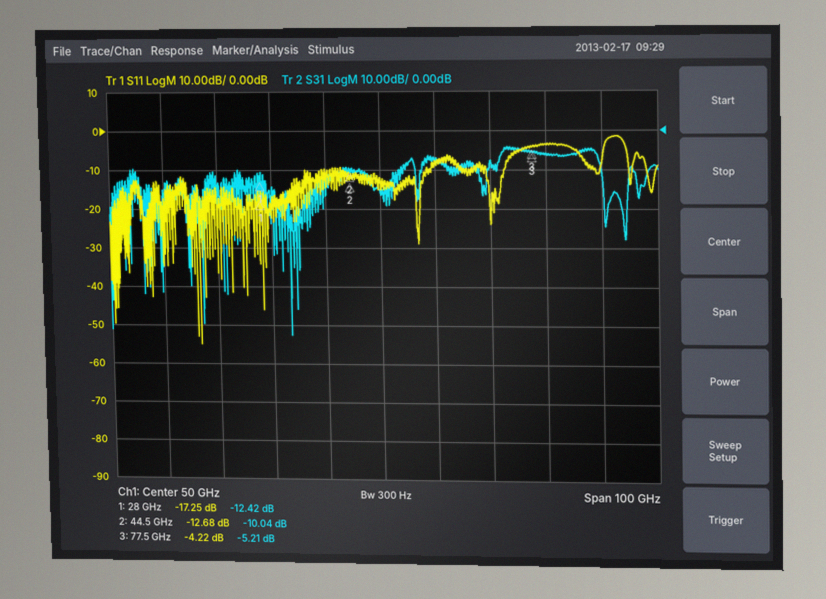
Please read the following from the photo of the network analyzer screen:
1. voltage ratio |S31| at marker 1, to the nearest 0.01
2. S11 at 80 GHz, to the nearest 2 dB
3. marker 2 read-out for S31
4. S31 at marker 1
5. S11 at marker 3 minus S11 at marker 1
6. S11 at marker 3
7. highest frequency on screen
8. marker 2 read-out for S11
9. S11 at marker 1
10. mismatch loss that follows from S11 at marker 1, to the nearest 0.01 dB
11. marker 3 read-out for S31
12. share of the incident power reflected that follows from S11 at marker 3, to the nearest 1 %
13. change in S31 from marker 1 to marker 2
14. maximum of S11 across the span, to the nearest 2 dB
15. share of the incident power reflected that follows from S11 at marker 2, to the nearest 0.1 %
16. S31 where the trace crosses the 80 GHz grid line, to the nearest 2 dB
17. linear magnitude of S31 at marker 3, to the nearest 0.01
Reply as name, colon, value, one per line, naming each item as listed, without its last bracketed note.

voltage ratio |S31| at marker 1, to the nearest 0.01: 0.24
S11 at 80 GHz, to the nearest 2 dB: -4 dB
marker 2 read-out for S31: -10.04 dB
S31 at marker 1: -12.42 dB
S11 at marker 3 minus S11 at marker 1: 13.03 dB
S11 at marker 3: -4.22 dB
highest frequency on screen: 100 GHz
marker 2 read-out for S11: -12.68 dB
S11 at marker 1: -17.25 dB
mismatch loss that follows from S11 at marker 1, to the nearest 0.01 dB: 0.08 dB
marker 3 read-out for S31: -5.21 dB
share of the incident power reflected that follows from S11 at marker 3, to the nearest 1 %: 38 %
change in S31 from marker 1 to marker 2: 2.38 dB
maximum of S11 across the span, to the nearest 2 dB: -2 dB
share of the incident power reflected that follows from S11 at marker 2, to the nearest 0.1 %: 5.4 %
S31 where the trace crosses the 80 GHz grid line, to the nearest 2 dB: -6 dB
linear magnitude of S31 at marker 3, to the nearest 0.01: 0.55
